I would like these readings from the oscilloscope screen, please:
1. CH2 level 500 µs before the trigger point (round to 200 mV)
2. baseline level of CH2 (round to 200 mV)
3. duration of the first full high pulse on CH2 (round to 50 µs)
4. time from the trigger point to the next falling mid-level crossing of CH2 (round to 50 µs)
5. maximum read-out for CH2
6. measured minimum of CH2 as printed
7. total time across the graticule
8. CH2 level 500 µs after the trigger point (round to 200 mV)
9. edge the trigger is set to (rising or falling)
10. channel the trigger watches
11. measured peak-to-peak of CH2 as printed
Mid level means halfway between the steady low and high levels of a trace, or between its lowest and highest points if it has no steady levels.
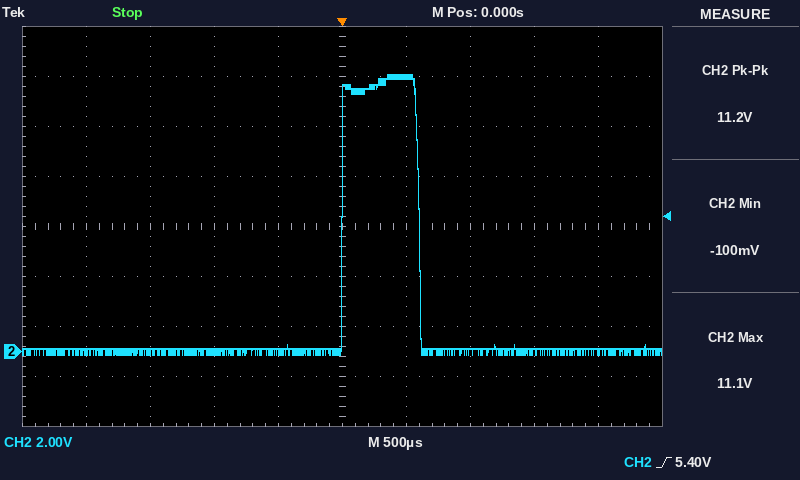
0.0 V
0.0 V
600 µs
600 µs
11.1 V
-100 mV
5 ms
11.0 V
rising
CH2
11.2 V
